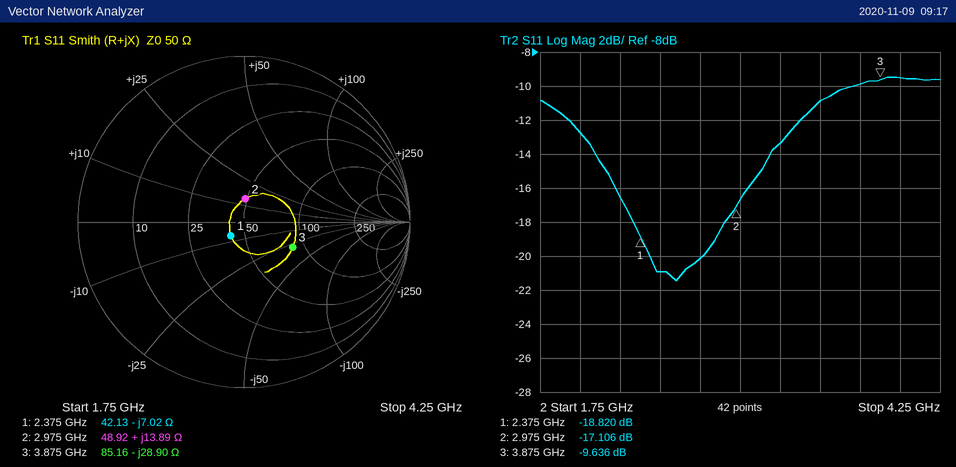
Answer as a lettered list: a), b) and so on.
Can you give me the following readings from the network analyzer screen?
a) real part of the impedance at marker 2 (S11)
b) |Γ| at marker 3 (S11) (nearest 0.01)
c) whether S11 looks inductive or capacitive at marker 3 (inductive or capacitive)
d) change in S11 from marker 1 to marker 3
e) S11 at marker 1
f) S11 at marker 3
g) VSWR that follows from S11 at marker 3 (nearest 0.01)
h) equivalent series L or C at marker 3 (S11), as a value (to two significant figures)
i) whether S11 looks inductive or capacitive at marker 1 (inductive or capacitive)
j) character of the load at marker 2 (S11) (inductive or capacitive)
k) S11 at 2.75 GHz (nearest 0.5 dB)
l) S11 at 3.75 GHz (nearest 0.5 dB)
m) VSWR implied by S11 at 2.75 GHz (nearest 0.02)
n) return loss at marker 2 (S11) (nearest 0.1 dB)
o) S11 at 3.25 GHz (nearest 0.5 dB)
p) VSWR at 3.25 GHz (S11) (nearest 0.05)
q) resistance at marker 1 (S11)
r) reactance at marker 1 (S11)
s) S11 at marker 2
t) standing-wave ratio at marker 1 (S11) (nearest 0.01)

a) 48.92 Ω
b) 0.33
c) capacitive
d) 9.184 dB
e) -18.820 dB
f) -9.636 dB
g) 1.98
h) 1.4 pF
i) capacitive
j) inductive
k) -20.0 dB
l) -10.0 dB
m) 1.22
n) 17.1 dB
o) -13.5 dB
p) 1.55
q) 42.13 Ω
r) -7.02 Ω
s) -17.106 dB
t) 1.26
